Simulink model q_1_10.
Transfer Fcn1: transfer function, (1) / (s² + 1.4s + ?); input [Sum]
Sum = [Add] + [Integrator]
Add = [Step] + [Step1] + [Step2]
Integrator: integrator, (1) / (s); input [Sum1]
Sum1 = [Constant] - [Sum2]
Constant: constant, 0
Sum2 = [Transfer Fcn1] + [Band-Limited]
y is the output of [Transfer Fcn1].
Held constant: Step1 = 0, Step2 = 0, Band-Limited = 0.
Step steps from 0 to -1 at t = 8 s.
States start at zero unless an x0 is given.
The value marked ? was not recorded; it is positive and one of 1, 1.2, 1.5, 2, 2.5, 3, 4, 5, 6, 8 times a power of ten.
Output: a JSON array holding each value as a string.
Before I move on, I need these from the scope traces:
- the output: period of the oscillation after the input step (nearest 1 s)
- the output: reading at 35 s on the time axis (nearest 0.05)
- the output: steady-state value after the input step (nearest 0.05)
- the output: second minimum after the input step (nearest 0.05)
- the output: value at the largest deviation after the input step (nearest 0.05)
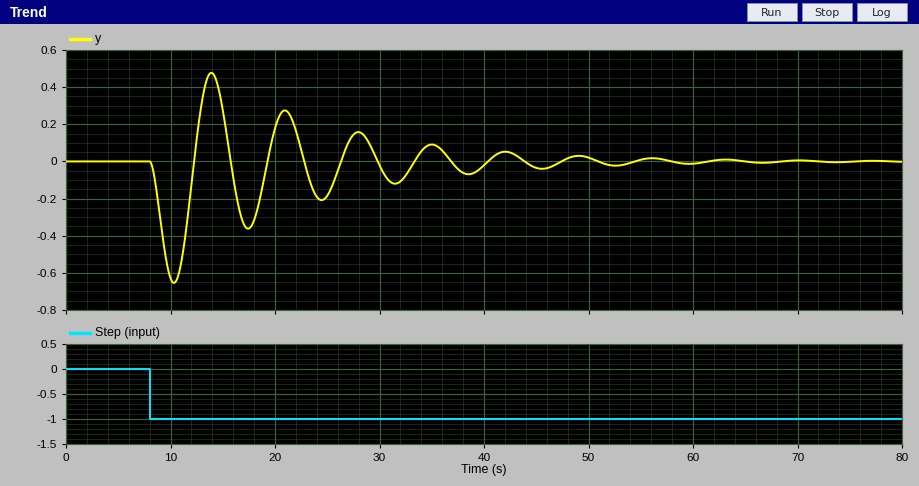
["7 s", "0.10", "0.00", "-0.35", "-0.65"]
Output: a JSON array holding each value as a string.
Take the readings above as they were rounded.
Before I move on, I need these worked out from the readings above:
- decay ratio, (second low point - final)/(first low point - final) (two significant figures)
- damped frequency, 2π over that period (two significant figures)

["0.54", "0.90 rad/s"]
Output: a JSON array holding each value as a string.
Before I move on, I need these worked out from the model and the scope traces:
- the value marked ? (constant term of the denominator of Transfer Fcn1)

["1"]
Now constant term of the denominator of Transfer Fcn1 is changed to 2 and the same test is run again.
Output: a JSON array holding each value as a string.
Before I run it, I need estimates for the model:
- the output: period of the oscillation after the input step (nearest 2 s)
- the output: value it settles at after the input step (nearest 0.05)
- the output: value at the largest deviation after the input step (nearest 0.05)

["6 s", "0.00", "-0.45"]
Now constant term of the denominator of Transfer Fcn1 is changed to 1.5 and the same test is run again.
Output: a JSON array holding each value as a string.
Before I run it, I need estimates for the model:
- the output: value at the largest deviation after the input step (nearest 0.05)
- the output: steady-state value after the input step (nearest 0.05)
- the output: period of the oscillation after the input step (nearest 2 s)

["-0.55", "0.00", "6 s"]
